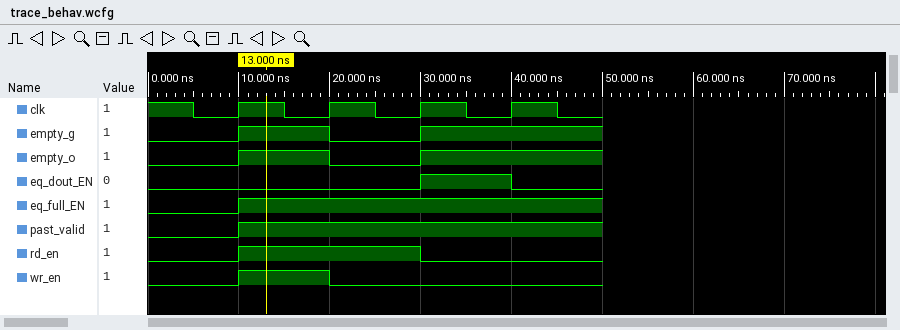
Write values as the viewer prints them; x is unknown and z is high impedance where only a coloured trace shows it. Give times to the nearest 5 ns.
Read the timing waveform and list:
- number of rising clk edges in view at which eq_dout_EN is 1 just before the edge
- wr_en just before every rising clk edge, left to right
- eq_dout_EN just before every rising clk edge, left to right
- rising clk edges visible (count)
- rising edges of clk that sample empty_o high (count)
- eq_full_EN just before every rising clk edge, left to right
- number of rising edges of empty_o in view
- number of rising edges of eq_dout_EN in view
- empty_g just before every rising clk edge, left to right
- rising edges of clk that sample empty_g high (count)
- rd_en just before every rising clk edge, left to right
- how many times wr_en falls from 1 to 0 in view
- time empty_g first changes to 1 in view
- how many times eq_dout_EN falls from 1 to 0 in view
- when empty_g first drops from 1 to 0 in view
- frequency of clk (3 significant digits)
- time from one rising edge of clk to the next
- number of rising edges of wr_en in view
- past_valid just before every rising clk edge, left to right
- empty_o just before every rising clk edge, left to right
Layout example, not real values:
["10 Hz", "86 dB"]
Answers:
["1", "0 1 0 0", "0 0 0 1", "4", "2", "0 1 1 1", "2", "1", "0 1 0 1", "2", "0 1 1 0", "1", "10 ns", "1", "20 ns", "100 MHz", "10 ns", "1", "0 1 1 1", "0 1 0 1"]
